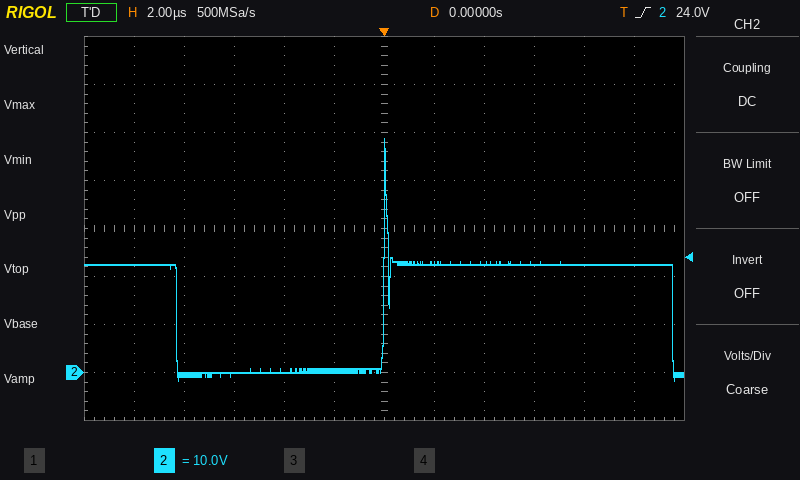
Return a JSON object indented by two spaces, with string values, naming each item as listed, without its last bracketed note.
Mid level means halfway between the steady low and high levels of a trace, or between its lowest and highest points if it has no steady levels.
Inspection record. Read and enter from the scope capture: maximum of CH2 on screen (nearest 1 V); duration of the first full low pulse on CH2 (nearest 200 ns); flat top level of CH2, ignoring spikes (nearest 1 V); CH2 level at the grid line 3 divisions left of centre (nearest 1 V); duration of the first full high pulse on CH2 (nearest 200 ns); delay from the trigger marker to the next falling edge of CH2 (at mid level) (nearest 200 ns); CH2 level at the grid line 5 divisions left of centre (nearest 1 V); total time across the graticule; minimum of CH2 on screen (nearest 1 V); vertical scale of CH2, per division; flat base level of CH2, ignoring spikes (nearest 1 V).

{
  "maximum of CH2 on screen": "49 V",
  "duration of the first full low pulse on CH2": "8.2 µs",
  "flat top level of CH2, ignoring spikes": "22 V",
  "CH2 level at the grid line 3 divisions left of centre": "0 V",
  "duration of the first full high pulse on CH2": "11.6 µs",
  "delay from the trigger marker to the next falling edge of CH2 (at mid level)": "11.6 µs",
  "CH2 level at the grid line 5 divisions left of centre": "22 V",
  "total time across the graticule": "24 µs",
  "minimum of CH2 on screen": "-2 V",
  "vertical scale of CH2, per division": "10 V",
  "flat base level of CH2, ignoring spikes": "0 V"
}
